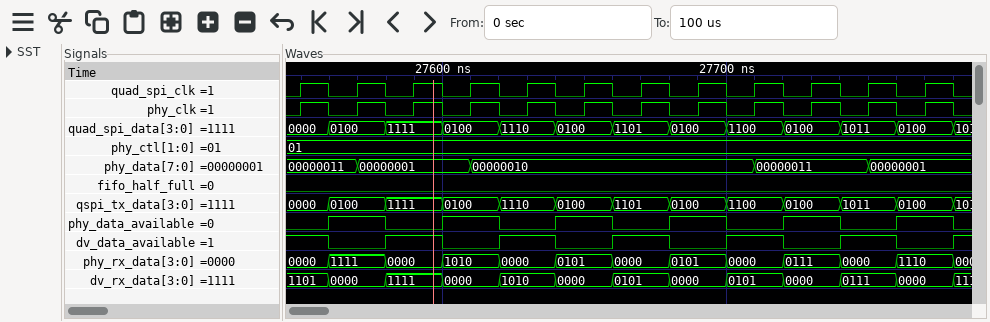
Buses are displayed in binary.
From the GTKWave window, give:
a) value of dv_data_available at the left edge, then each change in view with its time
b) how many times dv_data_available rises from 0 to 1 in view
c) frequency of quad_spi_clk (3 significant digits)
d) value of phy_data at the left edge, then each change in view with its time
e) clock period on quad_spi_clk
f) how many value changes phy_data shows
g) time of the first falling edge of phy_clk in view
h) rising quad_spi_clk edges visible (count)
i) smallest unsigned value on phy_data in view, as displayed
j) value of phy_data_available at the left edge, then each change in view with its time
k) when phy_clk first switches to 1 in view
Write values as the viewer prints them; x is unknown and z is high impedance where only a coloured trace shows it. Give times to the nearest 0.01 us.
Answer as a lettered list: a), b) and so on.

a) 1, 0 at 27.56 us, 1 at 27.58 us, 0 at 27.6 us, 1 at 27.62 us, 0 at 27.64 us, 1 at 27.66 us, 0 at 27.68 us, 1 at 27.7 us, 0 at 27.72 us, 1 at 27.74 us, 0 at 27.76 us, 1 at 27.78 us
b) 6
c) 50.0 MHz
d) 00000011, 00000001 at 27.57 us, 00000010 at 27.61 us, 00000011 at 27.71 us, 00000001 at 27.75 us
e) 0.02 us
f) 4
g) 27.56 us
h) 12
i) 00000001
j) 0, 1 at 27.56 us, 0 at 27.58 us, 1 at 27.6 us, 0 at 27.62 us, 1 at 27.64 us, 0 at 27.66 us, 1 at 27.68 us, 0 at 27.7 us, 1 at 27.72 us, 0 at 27.74 us, 1 at 27.76 us, 0 at 27.78 us
k) 27.55 us
